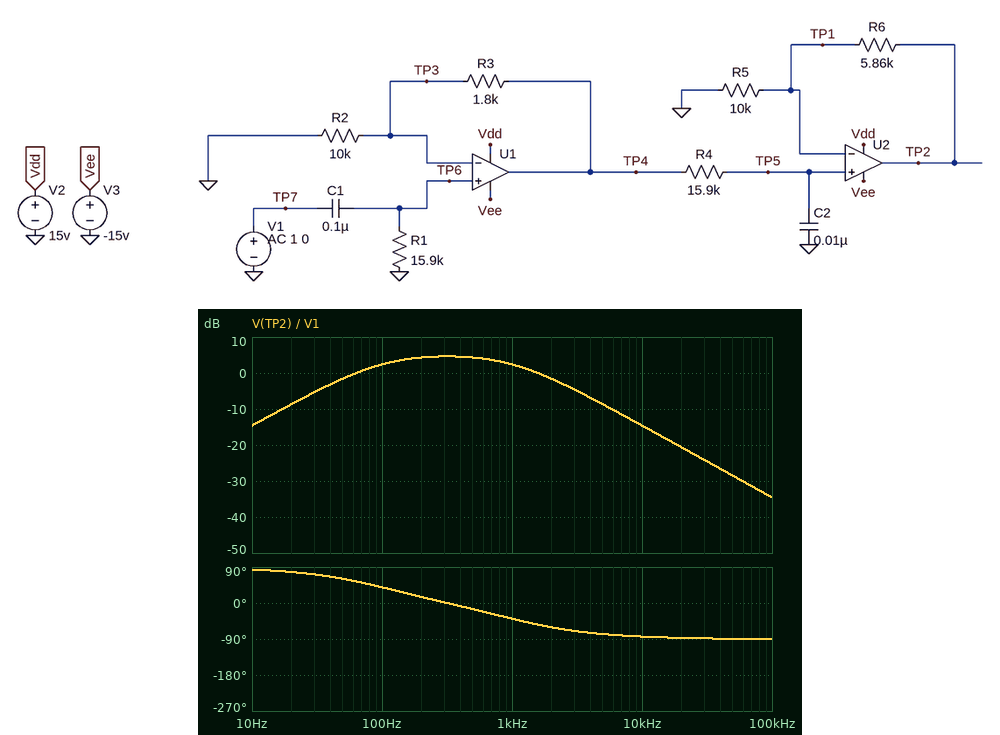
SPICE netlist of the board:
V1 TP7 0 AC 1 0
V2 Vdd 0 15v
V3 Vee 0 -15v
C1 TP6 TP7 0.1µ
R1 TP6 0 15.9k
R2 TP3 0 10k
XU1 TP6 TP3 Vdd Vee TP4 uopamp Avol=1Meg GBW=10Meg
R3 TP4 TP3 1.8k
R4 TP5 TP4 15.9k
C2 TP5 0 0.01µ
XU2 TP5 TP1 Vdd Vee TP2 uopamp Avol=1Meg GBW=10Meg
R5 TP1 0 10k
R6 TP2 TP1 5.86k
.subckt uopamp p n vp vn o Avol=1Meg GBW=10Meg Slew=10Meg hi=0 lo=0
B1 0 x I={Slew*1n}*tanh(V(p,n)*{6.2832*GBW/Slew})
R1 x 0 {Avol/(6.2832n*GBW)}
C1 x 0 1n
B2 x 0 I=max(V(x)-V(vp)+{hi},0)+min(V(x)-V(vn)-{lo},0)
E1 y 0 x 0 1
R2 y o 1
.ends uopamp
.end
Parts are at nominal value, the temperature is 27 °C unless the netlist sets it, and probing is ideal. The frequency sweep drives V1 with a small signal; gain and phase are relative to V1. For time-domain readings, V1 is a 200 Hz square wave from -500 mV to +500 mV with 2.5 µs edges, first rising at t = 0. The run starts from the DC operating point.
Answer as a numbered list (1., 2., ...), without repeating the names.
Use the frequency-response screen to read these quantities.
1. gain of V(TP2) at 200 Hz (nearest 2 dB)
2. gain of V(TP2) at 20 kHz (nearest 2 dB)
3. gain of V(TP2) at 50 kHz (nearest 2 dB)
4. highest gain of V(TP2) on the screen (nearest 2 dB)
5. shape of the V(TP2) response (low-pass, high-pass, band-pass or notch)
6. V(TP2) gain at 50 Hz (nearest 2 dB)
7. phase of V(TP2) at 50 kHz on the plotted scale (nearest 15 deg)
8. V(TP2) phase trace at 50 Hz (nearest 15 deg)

1. 4 dB
2. -20 dB
3. -28 dB
4. 4 dB
5. band-pass
6. -2 dB
7. -90 deg
8. 60 deg
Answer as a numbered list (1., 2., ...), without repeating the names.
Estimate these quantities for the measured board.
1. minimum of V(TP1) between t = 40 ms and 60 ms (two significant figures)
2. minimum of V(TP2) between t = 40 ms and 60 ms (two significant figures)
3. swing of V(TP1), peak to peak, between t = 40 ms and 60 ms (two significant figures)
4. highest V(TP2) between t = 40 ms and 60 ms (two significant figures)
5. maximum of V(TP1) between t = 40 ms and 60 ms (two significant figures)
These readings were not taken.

1. -740 mV
2. -1.2 V
3. 1.5 V
4. 1.2 V
5. 740 mV
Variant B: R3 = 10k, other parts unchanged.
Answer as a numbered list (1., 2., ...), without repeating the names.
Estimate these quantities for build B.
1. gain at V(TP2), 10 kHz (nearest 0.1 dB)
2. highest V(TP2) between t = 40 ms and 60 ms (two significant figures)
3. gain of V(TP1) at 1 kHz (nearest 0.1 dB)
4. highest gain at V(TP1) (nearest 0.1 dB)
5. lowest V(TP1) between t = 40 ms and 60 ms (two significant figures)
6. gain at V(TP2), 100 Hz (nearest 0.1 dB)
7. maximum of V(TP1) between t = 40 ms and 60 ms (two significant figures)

1. -10.0 dB
2. 2.0 V
3. 3.0 dB
4. 5.2 dB
5. -1.3 V
6. 7.0 dB
7. 1.3 V
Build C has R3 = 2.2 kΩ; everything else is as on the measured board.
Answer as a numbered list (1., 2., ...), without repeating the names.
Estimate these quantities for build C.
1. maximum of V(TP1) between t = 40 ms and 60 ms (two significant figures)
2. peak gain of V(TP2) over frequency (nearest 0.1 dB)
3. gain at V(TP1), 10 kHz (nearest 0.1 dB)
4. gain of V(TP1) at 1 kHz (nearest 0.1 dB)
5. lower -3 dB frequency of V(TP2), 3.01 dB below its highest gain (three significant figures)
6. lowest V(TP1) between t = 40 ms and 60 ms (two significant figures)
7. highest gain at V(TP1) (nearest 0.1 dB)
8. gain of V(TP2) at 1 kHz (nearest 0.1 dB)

1. 770 mV
2. 4.9 dB
3. -18.3 dB
4. -1.3 dB
5. 84.5 Hz
6. -770 mV
7. 0.9 dB
8. 2.7 dB
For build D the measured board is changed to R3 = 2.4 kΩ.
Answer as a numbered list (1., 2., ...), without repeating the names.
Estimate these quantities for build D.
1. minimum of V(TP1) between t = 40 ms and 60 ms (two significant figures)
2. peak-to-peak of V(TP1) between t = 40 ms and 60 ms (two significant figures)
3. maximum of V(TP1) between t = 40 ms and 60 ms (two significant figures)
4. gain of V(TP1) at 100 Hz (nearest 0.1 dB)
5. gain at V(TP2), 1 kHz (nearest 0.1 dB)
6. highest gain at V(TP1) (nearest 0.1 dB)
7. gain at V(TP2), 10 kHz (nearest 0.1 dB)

1. -780 mV
2. 1.6 V
3. 780 mV
4. -1.2 dB
5. 2.8 dB
6. 1.0 dB
7. -14.2 dB
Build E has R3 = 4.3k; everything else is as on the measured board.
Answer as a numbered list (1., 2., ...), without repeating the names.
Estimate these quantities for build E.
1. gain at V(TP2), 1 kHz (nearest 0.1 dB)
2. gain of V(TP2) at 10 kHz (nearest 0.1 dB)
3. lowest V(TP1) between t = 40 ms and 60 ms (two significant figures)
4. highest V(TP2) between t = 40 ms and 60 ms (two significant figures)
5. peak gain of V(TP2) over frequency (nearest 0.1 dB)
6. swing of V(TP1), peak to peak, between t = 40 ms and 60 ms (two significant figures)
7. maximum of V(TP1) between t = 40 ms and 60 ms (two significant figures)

1. 4.1 dB
2. -12.9 dB
3. -900 mV
4. 1.4 V
5. 6.3 dB
6. 1.8 V
7. 900 mV
